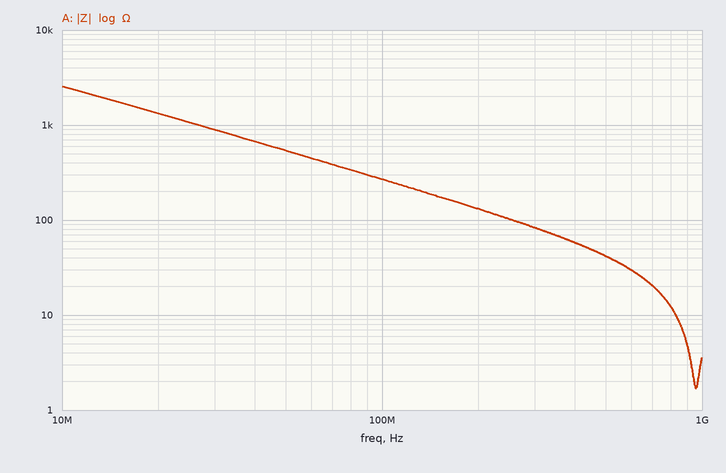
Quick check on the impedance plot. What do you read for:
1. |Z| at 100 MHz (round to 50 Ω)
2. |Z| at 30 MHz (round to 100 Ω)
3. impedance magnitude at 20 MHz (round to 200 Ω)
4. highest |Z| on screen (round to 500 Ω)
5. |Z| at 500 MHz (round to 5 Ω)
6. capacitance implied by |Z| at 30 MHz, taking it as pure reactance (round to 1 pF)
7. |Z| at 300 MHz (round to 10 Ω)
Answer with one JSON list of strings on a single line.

["250 Ω", "900 Ω", "1.4 kΩ", "2.5 kΩ", "40 Ω", "6 pF", "80 Ω"]
